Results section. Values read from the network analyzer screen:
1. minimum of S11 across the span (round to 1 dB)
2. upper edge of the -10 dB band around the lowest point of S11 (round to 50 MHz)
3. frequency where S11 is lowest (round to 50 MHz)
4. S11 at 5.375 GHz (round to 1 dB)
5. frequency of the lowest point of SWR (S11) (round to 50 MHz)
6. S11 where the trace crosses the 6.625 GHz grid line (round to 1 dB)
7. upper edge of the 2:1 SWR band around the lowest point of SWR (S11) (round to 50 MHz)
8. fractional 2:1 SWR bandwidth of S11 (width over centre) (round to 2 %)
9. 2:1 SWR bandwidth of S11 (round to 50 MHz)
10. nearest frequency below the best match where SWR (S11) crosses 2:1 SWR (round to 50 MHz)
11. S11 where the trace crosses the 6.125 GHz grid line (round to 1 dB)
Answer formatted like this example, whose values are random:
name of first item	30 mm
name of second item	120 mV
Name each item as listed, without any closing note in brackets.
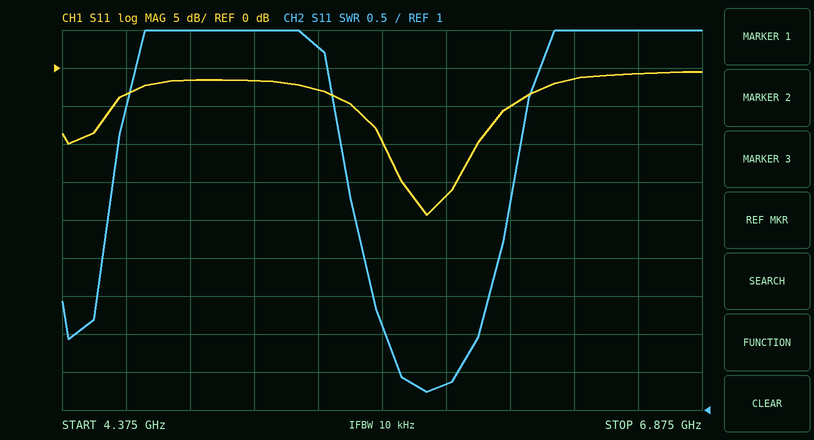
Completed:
minimum of S11 across the span	-19 dB
upper edge of the -10 dB band around the lowest point of S11	6.00 GHz
frequency where S11 is lowest	5.80 GHz
S11 at 5.375 GHz	-3 dB
frequency of the lowest point of SWR (S11)	5.80 GHz
S11 where the trace crosses the 6.625 GHz grid line	-1 dB
upper edge of the 2:1 SWR band around the lowest point of SWR (S11)	6.00 GHz
fractional 2:1 SWR bandwidth of S11 (width over centre)	6 %
2:1 SWR bandwidth of S11	350 MHz
nearest frequency below the best match where SWR (S11) crosses 2:1 SWR	5.65 GHz
S11 where the trace crosses the 6.125 GHz grid line	-5 dB
